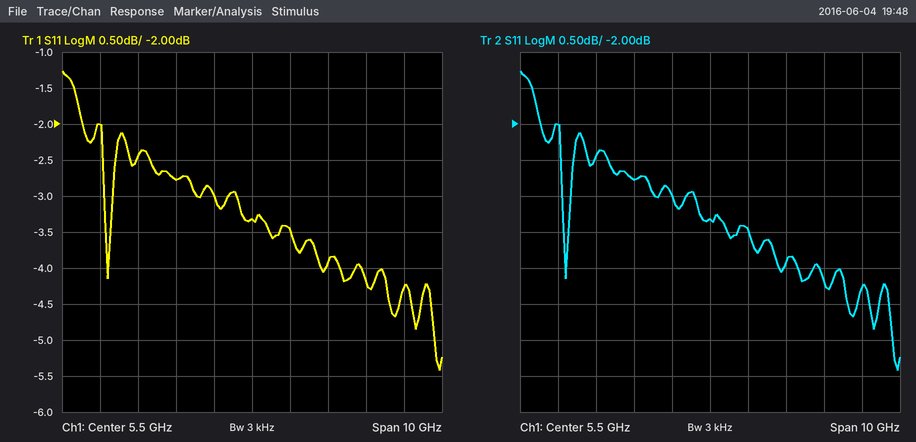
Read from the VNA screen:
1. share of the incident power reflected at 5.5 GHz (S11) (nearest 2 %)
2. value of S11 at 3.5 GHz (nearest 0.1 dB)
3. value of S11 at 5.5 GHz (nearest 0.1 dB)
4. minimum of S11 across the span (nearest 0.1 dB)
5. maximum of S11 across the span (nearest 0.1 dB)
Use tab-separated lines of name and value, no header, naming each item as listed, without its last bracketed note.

share of the incident power reflected at 5.5 GHz (S11)	46 %
value of S11 at 3.5 GHz	-2.8 dB
value of S11 at 5.5 GHz	-3.3 dB
minimum of S11 across the span	-5.4 dB
maximum of S11 across the span	-1.3 dB
